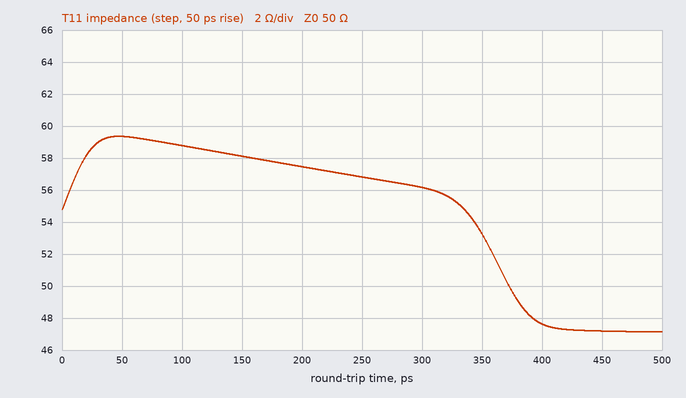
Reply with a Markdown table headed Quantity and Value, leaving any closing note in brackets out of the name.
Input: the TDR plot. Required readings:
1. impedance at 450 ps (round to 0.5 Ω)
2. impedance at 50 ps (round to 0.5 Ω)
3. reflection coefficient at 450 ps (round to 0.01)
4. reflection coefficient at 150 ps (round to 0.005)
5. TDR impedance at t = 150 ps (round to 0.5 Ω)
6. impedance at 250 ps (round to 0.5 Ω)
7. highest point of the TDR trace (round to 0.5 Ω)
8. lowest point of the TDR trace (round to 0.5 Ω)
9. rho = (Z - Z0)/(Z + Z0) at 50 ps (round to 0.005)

| Quantity | Value |
|---|---|
| impedance at 450 ps | 47.0 Ω |
| impedance at 50 ps | 59.5 Ω |
| reflection coefficient at 450 ps | -0.03 |
| reflection coefficient at 150 ps | +0.075 |
| TDR impedance at t = 150 ps | 58.0 Ω |
| impedance at 250 ps | 57.0 Ω |
| highest point of the TDR trace | 59.5 Ω |
| lowest point of the TDR trace | 47.0 Ω |
| rho = (Z - Z0)/(Z + Z0) at 50 ps | +0.085 |
